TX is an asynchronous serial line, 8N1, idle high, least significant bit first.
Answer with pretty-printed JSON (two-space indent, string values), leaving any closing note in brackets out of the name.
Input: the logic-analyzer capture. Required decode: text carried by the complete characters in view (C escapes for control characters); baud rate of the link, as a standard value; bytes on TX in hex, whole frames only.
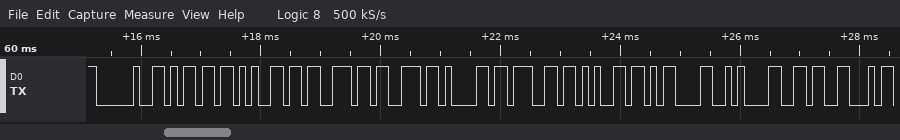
{
  "text carried by the complete characters in view": "\" message\\r\\n6\"",
  "baud rate of the link, as a standard value": "9600 baud",
  "bytes on TX in hex, whole frames only": "0x20 0x6D 0x65 0x73 0x73 0x61 0x67 0x65 0x0D 0x0A 0x36"
}
